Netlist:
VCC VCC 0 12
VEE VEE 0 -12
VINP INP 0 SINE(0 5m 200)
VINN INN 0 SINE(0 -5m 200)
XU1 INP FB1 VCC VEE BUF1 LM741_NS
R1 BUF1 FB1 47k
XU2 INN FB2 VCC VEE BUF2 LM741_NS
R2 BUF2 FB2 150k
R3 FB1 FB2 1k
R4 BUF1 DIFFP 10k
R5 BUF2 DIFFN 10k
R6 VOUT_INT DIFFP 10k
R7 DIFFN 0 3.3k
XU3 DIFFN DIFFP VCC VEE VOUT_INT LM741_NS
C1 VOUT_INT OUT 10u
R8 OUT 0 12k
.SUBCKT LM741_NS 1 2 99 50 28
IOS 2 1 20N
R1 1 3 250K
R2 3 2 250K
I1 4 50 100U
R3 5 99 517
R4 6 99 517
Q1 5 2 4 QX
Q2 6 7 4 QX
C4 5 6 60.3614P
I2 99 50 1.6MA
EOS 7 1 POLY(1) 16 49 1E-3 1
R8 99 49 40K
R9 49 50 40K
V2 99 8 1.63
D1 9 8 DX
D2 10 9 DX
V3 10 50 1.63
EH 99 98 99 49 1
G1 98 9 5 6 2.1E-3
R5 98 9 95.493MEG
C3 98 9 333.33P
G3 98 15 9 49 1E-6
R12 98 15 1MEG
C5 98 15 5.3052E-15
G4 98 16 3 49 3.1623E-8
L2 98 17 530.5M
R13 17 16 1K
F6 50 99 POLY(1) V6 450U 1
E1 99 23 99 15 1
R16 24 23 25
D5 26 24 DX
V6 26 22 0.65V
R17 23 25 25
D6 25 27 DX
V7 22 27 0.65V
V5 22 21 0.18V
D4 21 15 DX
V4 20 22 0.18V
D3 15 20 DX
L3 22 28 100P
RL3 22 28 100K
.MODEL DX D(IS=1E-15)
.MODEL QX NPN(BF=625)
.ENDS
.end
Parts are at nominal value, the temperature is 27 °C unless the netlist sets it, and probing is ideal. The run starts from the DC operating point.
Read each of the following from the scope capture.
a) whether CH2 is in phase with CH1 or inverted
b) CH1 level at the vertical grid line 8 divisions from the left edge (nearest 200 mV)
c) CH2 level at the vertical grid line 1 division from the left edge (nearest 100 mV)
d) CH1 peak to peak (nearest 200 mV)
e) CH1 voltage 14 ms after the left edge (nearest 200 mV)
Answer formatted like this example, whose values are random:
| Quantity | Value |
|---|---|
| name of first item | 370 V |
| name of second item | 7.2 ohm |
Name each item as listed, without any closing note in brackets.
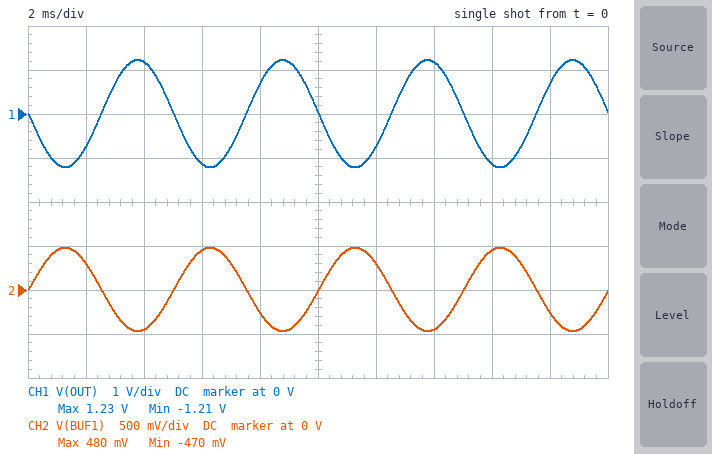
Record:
| Quantity | Value |
|---|---|
| whether CH2 is in phase with CH1 or inverted | inverted |
| CH1 level at the vertical grid line 8 divisions from the left edge | -1.2 V |
| CH2 level at the vertical grid line 1 division from the left edge | 300 mV |
| CH1 peak to peak | 2.4 V |
| CH1 voltage 14 ms after the left edge | 1.2 V |
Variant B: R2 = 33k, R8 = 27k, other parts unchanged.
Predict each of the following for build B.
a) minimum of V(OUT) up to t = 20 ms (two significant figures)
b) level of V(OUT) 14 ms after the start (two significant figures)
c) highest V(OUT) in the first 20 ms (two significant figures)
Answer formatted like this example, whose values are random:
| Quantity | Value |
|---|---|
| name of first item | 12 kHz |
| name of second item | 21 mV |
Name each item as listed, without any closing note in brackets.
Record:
| Quantity | Value |
|---|---|
| minimum of V(OUT) up to t = 20 ms | -640 mV |
| level of V(OUT) 14 ms after the start | 610 mV |
| highest V(OUT) in the first 20 ms | 640 mV |
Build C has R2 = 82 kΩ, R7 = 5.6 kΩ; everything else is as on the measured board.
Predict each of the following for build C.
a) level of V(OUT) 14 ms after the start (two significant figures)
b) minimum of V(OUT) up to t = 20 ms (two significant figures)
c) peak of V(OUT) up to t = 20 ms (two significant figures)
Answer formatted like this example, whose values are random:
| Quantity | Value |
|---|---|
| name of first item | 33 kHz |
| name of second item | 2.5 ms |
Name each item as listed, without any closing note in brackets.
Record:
| Quantity | Value |
|---|---|
| level of V(OUT) 14 ms after the start | 1.0 V |
| minimum of V(OUT) up to t = 20 ms | -1.1 V |
| peak of V(OUT) up to t = 20 ms | 1.1 V |
